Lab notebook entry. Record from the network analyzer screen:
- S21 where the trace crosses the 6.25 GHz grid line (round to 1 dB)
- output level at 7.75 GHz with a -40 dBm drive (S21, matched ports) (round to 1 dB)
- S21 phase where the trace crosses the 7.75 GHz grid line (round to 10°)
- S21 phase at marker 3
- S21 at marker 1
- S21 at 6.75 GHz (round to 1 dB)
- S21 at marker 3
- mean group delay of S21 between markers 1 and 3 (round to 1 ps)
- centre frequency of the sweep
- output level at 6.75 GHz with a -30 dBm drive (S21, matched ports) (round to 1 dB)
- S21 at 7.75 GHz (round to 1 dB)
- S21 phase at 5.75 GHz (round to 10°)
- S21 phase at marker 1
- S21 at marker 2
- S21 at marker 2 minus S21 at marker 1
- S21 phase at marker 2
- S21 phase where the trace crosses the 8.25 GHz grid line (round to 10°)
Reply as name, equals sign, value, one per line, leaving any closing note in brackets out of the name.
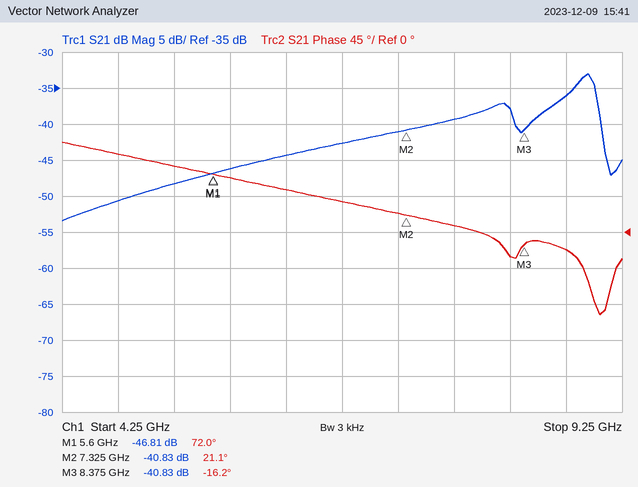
S21 where the trace crosses the 6.25 GHz grid line = -44 dB
output level at 7.75 GHz with a -40 dBm drive (S21, matched ports) = -79 dBm
S21 phase where the trace crosses the 7.75 GHz grid line = 10°
S21 phase at marker 3 = -16.2°
S21 at marker 1 = -46.81 dB
S21 at 6.75 GHz = -43 dB
S21 at marker 3 = -40.83 dB
mean group delay of S21 between markers 1 and 3 = 88 ps
centre frequency of the sweep = 6.75 GHz
output level at 6.75 GHz with a -30 dBm drive (S21, matched ports) = -73 dBm
S21 at 7.75 GHz = -39 dB
S21 phase at 5.75 GHz = 70°
S21 phase at marker 1 = 72.0°
S21 at marker 2 = -40.83 dB
S21 at marker 2 minus S21 at marker 1 = 5.98 dB
S21 phase at marker 2 = 21.1°
S21 phase where the trace crosses the 8.25 GHz grid line = -30°
